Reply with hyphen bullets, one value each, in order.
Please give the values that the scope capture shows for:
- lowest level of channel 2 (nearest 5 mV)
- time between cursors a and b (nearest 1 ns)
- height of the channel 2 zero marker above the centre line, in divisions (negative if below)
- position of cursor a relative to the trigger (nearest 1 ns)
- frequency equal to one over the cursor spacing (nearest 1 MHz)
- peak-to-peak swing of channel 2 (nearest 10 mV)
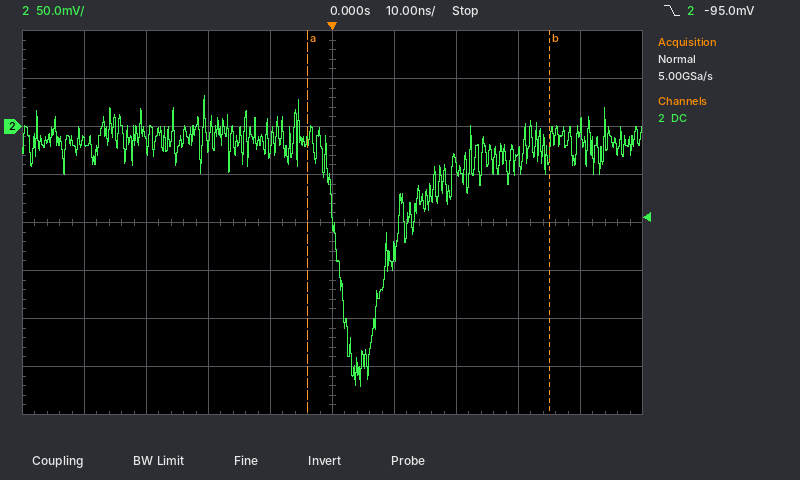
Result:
- -270 mV
- 39 ns
- +2.0 div
- -4 ns
- 26 MHz
- 300 mV
